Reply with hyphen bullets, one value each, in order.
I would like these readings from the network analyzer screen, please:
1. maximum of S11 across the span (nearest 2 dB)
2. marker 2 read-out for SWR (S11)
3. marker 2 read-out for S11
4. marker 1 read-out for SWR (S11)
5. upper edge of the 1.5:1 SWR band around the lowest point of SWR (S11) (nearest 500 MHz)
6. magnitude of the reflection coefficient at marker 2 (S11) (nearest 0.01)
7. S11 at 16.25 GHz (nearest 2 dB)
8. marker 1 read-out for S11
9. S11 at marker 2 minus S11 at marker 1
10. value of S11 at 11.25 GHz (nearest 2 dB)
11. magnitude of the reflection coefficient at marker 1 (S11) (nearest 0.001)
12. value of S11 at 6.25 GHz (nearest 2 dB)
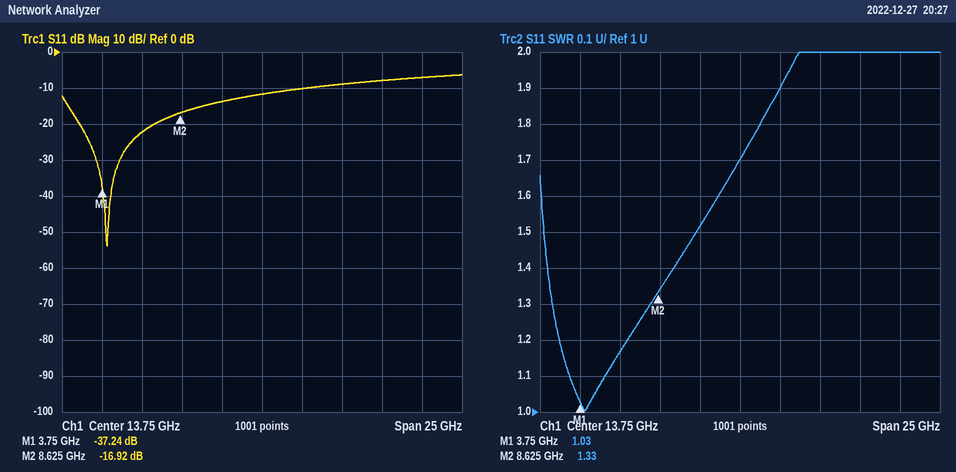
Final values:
- -6 dB
- 1.33
- -16.92 dB
- 1.03
- 11.0 GHz
- 0.14
- -10 dB
- -37.24 dB
- 20.32 dB
- -14 dB
- 0.014
- -22 dB
